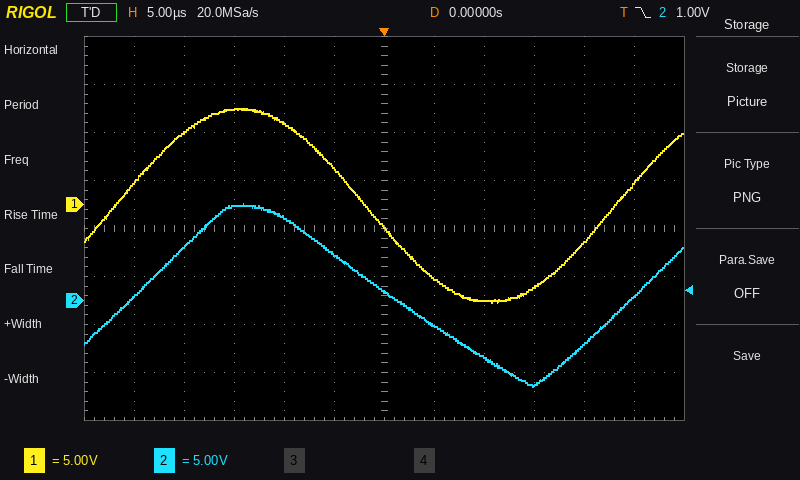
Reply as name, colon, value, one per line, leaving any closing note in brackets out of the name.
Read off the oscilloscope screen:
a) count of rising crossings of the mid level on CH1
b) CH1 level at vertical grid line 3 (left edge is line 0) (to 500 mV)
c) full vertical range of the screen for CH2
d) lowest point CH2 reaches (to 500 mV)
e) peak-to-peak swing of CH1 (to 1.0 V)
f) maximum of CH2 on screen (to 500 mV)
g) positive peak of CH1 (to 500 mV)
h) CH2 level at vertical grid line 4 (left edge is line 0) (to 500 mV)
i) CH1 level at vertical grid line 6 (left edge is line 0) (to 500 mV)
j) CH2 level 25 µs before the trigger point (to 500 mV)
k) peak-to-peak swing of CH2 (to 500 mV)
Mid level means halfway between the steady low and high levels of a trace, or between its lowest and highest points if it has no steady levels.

count of rising crossings of the mid level on CH1: 2
CH1 level at vertical grid line 3 (left edge is line 0): 10.0 V
full vertical range of the screen for CH2: 40 V
lowest point CH2 reaches: -9.0 V
peak-to-peak swing of CH1: 20.0 V
maximum of CH2 on screen: 10.0 V
positive peak of CH1: 10.0 V
CH2 level at vertical grid line 4 (left edge is line 0): 8.5 V
CH1 level at vertical grid line 6 (left edge is line 0): -2.5 V
CH2 level 25 µs before the trigger point: 500 mV
peak-to-peak swing of CH2: 19.0 V
